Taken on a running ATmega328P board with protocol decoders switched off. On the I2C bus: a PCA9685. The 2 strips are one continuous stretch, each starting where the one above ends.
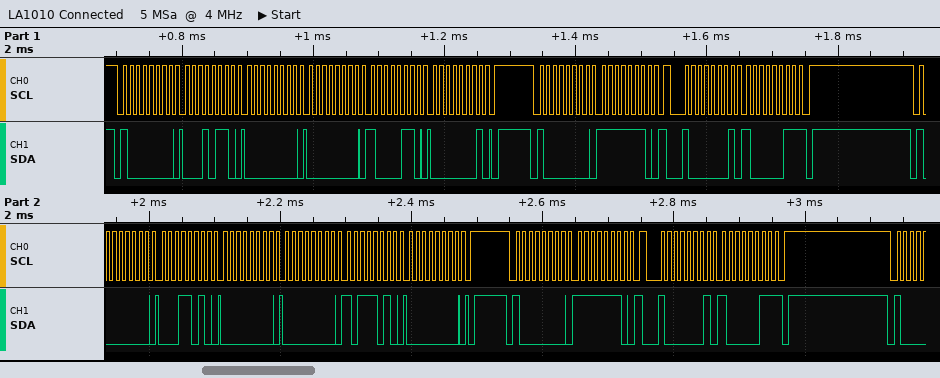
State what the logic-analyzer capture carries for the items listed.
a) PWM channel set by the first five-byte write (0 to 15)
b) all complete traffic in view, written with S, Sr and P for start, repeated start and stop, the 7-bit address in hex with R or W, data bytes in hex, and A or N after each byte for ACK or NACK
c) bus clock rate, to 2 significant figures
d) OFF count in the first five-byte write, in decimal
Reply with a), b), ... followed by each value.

a) 4
b) S 40W A 16 A 00 A 00 A 86 A 01 A P S 40W A FE A Sr 40R A 83 N P S 40W A 1A A 00 A 00 A BA A 00 A P S 40W A FE A Sr 40R A 83 N P
c) 100 kHz
d) 390
